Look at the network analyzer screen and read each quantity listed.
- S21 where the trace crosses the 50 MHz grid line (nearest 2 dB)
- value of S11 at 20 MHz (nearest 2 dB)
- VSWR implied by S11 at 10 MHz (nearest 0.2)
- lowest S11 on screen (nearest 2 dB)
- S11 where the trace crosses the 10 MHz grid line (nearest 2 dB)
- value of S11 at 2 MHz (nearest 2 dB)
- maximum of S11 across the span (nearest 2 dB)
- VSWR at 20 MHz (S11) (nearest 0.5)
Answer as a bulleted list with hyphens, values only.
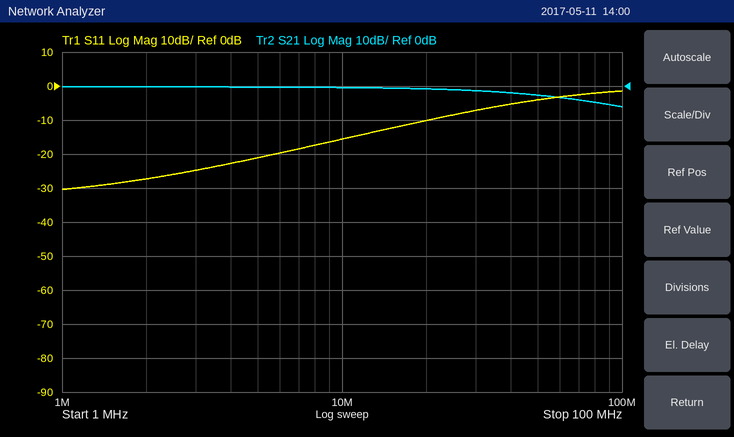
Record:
- -2 dB
- -10 dB
- 1.4
- -30 dB
- -16 dB
- -28 dB
- -2 dB
- 2.0
